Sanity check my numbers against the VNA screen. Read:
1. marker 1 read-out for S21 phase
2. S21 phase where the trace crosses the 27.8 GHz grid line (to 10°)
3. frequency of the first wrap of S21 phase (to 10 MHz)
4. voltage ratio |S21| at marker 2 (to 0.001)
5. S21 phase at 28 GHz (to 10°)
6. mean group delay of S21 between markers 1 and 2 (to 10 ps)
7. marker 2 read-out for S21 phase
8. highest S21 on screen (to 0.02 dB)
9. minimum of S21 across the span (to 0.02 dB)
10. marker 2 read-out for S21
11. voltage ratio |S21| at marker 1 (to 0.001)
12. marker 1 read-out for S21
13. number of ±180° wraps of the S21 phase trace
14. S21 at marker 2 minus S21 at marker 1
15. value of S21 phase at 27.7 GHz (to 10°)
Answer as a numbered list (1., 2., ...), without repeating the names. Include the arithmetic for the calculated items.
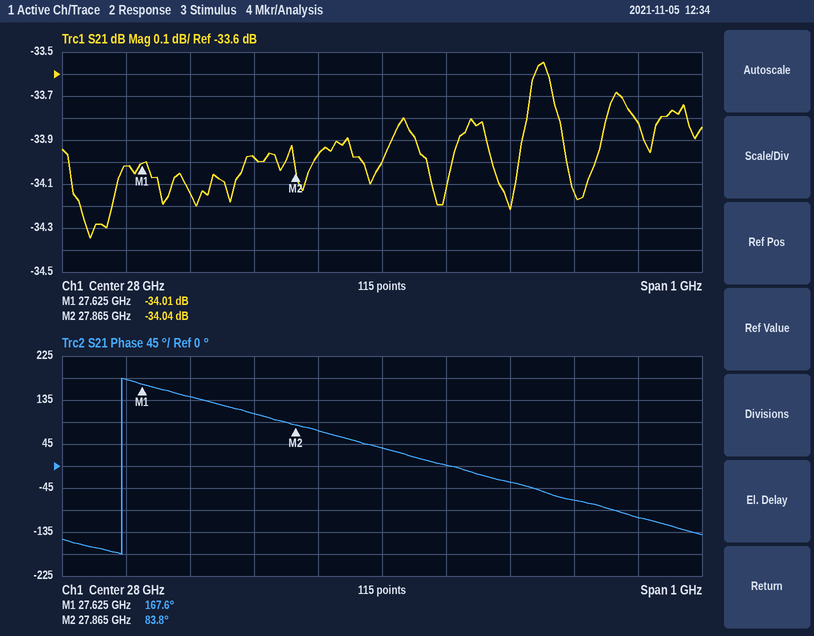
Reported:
1. 167.6°
2. 110°
3. 27.59 GHz
4. 10^(-34.04/20) ≈ 0.020
5. 40°
6. −(83.8° − (167.6°))/(360° × 240 MHz) ≈ 970 ps
7. 83.8°
8. -33.54 dB
9. -34.34 dB
10. -34.04 dB
11. 10^(-34.01/20) ≈ 0.020
12. -34.01 dB
13. 1
14. -34.04 − (-34.01) = -0.03 dB
15. 140°
